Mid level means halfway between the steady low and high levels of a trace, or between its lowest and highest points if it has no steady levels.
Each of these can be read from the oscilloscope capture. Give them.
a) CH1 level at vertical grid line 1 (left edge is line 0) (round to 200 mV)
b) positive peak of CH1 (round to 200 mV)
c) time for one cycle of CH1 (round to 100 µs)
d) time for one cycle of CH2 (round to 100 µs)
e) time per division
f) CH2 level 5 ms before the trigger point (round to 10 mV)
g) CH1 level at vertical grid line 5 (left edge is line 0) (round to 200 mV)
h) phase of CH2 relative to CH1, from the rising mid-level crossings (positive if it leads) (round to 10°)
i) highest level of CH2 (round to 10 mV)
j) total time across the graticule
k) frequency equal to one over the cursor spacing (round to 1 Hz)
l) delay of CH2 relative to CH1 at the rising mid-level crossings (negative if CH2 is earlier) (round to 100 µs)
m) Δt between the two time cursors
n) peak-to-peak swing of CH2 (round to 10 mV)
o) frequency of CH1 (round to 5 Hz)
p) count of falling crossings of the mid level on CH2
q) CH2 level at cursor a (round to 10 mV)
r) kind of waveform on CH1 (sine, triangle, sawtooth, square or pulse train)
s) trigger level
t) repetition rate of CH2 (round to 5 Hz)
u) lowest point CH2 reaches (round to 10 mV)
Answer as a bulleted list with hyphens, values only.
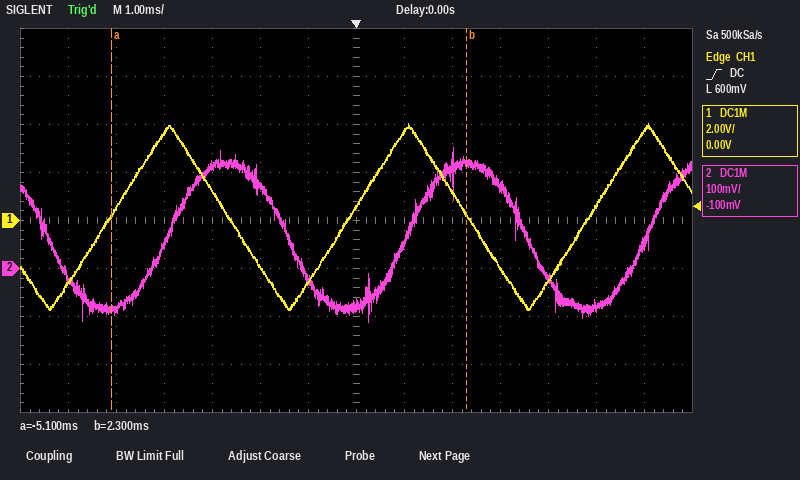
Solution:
- -2.6 V
- 4.0 V
- 5.0 ms
- 5.0 ms
- 1 ms
- -90 mV
- -2.0 V
- -90°
- 250 mV
- 14 ms
- 135 Hz
- +1.2 ms
- 7.4 ms
- 360 mV
- 200 Hz
- 3
- -90 mV
- triangle
- 600 mV
- 200 Hz
- -110 mV
